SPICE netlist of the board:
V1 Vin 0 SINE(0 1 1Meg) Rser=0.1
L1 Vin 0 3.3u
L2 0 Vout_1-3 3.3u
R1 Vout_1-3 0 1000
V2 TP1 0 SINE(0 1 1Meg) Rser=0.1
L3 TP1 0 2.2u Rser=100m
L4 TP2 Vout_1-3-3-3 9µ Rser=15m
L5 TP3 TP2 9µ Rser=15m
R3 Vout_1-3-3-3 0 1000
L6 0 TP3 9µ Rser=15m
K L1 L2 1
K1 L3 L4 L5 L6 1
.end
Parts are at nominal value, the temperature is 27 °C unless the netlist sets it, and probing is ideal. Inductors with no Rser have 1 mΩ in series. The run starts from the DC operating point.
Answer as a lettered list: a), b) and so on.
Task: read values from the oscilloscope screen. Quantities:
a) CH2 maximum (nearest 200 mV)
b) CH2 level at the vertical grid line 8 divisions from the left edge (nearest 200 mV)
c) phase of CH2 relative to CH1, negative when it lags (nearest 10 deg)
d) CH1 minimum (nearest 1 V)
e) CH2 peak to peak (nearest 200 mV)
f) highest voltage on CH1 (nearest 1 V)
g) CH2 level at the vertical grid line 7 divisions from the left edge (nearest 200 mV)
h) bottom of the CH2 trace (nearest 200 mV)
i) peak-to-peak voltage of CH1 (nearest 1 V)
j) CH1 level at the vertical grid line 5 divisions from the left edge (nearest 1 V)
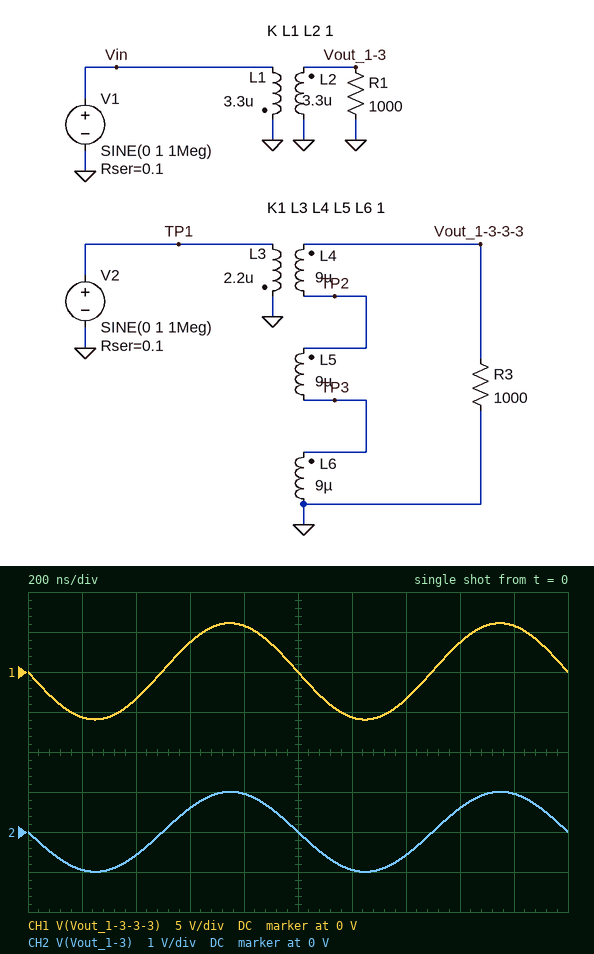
a) 1.0 V
b) 600 mV
c) 0 deg
d) -6 V
e) 2.0 V
f) 6 V
g) -600 mV
h) -1.0 V
i) 12 V
j) 0 V
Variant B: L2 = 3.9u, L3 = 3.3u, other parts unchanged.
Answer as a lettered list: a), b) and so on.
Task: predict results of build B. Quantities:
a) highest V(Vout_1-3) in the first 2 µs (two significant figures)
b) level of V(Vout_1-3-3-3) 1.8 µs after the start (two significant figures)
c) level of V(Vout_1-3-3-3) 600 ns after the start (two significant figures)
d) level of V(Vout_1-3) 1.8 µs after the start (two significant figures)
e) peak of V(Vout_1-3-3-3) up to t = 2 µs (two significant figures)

a) 1.1 V
b) 4.7 V
c) 3.0 V
d) 1.0 V
e) 5.0 V
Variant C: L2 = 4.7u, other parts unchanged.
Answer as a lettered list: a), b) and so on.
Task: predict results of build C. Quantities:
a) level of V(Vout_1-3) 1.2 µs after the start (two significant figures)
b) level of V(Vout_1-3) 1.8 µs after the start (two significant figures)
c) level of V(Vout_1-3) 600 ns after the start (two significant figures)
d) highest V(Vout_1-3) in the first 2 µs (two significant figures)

a) -1.1 V
b) 1.1 V
c) 710 mV
d) 1.2 V
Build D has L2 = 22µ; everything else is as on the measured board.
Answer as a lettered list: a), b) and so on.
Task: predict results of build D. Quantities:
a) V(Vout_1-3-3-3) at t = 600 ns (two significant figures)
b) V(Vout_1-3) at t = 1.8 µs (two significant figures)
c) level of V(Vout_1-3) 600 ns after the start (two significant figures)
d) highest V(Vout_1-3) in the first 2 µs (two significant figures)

a) 3.7 V
b) 2.5 V
c) 1.5 V
d) 2.6 V
